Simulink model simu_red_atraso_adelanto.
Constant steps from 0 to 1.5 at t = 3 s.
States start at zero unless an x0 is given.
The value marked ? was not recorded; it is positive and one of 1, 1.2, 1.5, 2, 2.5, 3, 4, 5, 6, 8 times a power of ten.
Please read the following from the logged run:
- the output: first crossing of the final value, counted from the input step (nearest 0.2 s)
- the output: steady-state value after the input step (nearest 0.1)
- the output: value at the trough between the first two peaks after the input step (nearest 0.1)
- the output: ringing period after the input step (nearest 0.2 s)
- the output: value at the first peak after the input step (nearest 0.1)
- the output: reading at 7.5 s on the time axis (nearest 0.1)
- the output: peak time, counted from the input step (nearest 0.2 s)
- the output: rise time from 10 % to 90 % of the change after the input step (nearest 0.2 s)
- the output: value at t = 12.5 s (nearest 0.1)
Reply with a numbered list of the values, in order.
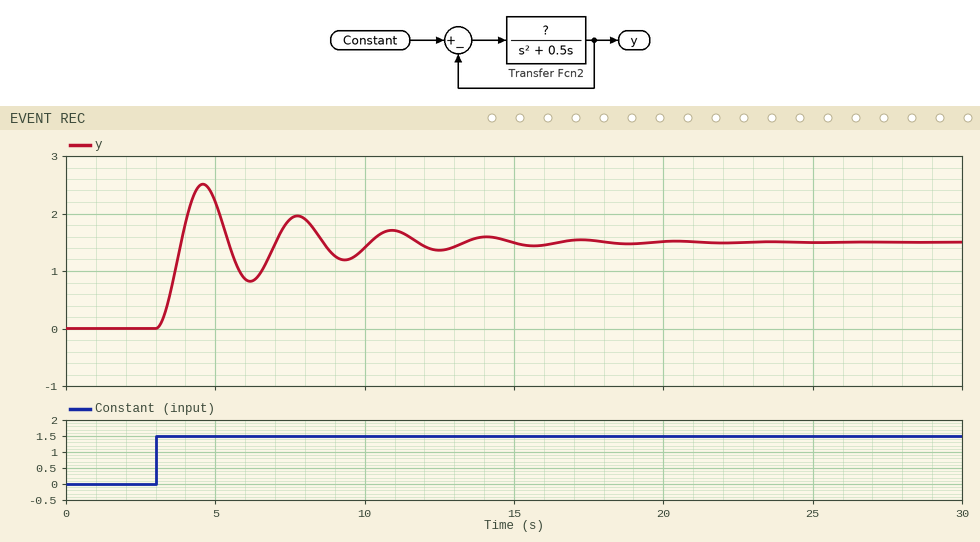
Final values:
1. 0.8 s
2. 1.5
3. 0.8
4. 3.2 s
5. 2.5
6. 1.9
7. 1.6 s
8. 0.6 s
9. 1.4
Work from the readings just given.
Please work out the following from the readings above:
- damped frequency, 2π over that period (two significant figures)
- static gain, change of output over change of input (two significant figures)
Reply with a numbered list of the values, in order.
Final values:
1. 2.0 rad/s
2. 1.0
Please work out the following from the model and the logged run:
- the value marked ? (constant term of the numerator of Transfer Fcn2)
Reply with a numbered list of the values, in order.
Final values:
1. 4
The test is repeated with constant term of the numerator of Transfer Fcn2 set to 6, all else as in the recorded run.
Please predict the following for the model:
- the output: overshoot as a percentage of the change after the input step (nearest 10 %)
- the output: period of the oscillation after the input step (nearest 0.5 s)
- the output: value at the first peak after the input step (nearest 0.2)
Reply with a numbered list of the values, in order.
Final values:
1. 70 %
2. 2.5 s
3. 2.6
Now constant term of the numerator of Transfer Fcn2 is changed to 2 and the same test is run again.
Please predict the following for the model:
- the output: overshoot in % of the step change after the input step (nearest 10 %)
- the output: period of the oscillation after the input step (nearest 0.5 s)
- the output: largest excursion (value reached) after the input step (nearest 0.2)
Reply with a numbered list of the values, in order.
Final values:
1. 60 %
2. 4.5 s
3. 2.4
